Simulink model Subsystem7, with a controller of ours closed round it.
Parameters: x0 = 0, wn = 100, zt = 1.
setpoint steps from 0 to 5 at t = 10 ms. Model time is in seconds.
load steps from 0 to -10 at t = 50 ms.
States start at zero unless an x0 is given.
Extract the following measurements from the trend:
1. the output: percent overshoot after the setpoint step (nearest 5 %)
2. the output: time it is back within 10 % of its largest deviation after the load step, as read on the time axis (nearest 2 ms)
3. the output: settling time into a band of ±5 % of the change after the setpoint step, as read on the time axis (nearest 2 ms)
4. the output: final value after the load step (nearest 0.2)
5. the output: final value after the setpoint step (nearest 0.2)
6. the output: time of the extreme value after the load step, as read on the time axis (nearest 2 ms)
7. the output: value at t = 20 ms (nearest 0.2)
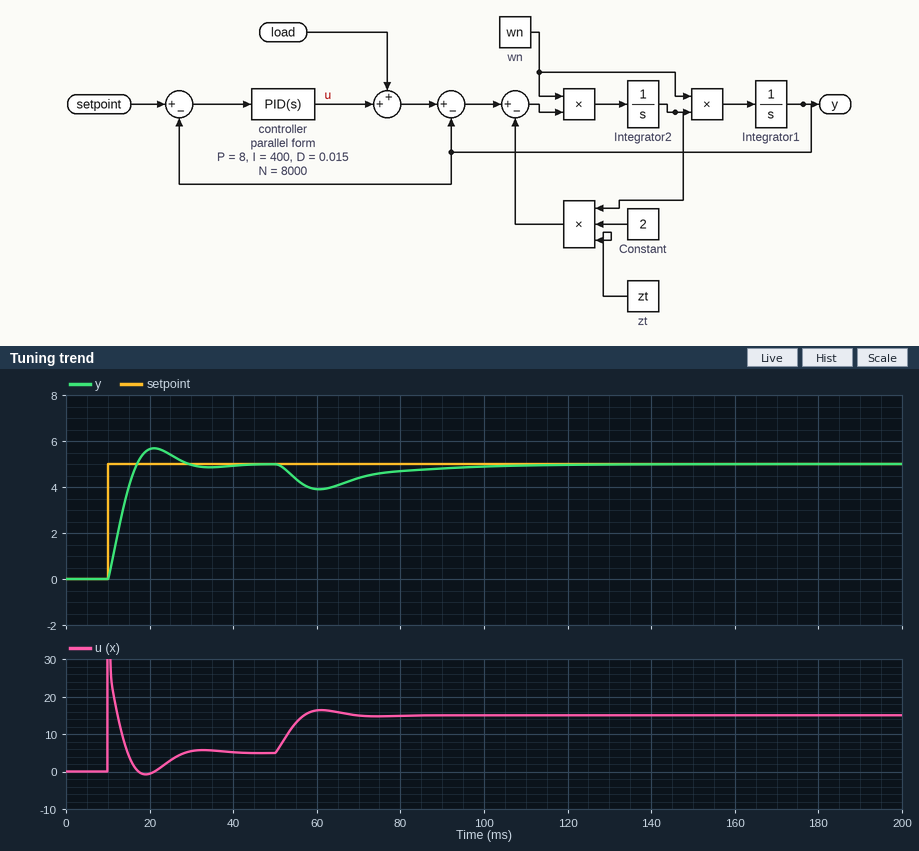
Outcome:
15 %
100 ms
26 ms
5.0
5.0
60 ms
5.6
